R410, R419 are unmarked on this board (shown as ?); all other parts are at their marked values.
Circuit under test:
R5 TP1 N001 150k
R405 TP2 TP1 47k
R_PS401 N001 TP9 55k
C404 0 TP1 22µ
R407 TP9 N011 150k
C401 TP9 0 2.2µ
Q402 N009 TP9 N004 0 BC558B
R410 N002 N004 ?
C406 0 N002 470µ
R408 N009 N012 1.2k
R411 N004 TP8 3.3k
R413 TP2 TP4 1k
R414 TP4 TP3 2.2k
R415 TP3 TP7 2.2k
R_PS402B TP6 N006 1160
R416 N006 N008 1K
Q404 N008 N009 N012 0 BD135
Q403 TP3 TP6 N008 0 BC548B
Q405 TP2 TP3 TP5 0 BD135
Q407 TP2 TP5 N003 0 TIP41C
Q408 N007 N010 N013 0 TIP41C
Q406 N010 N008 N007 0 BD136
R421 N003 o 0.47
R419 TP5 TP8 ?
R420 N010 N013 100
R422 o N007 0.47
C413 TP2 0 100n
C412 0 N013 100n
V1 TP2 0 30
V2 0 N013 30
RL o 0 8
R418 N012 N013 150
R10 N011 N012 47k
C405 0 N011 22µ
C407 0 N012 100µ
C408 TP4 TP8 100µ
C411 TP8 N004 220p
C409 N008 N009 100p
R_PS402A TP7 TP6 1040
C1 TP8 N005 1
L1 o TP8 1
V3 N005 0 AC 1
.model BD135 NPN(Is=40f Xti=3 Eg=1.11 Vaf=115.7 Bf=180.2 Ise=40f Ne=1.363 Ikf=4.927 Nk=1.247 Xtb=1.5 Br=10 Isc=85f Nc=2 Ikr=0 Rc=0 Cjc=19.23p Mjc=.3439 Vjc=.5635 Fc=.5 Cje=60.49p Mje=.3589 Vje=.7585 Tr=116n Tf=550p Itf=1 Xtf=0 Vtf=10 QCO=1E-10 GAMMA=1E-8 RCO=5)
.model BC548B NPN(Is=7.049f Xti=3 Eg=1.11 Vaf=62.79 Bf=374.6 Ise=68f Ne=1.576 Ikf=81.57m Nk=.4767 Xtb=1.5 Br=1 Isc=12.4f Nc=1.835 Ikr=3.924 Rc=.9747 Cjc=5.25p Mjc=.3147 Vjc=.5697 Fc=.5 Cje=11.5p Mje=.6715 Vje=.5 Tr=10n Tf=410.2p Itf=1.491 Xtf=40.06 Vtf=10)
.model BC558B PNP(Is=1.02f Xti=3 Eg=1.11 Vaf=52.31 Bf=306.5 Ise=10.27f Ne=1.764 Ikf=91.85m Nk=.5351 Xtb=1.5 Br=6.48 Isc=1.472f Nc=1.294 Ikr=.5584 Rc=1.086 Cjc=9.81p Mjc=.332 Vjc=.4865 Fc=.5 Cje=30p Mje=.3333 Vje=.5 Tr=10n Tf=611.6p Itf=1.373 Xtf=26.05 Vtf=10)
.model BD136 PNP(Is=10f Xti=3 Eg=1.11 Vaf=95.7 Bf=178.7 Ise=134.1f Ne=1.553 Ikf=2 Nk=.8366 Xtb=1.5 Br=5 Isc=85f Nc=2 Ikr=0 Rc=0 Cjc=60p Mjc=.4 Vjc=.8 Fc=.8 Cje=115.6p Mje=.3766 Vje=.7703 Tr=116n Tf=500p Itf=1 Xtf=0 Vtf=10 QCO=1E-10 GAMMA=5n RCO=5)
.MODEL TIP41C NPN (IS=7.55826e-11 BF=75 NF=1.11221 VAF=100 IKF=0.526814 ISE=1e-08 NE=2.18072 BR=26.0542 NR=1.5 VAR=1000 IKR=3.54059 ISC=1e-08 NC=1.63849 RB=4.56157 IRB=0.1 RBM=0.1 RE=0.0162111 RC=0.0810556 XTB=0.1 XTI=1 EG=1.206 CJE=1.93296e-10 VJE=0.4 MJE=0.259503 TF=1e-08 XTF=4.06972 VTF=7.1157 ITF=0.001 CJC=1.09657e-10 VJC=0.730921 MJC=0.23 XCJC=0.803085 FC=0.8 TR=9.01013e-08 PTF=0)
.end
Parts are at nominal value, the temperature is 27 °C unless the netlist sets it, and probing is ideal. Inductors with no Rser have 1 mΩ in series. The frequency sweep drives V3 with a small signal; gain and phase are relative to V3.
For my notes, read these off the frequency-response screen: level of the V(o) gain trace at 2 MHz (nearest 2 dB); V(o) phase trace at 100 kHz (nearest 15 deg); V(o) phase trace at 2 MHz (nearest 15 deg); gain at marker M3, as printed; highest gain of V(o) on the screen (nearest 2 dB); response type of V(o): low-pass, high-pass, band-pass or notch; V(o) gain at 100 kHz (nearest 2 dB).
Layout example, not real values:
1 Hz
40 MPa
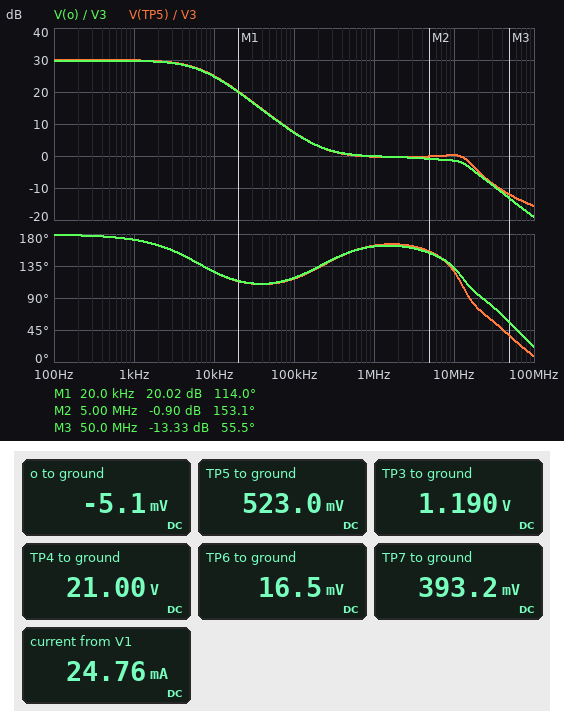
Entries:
0 dB
120 deg
165 deg
-13.33 dB
30 dB
low-pass
8 dB
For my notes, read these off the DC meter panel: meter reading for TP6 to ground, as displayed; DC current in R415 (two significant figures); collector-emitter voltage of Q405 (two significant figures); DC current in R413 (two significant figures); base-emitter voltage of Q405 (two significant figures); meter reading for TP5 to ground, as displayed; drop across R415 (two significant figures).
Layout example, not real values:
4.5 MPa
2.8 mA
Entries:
16.5 mV
360 µA
29 V
9.0 mA
670 mV
523.0 mV
800 mV
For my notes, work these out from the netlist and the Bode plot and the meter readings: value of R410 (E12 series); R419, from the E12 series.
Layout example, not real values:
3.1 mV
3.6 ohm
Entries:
47 Ω
68 Ω
